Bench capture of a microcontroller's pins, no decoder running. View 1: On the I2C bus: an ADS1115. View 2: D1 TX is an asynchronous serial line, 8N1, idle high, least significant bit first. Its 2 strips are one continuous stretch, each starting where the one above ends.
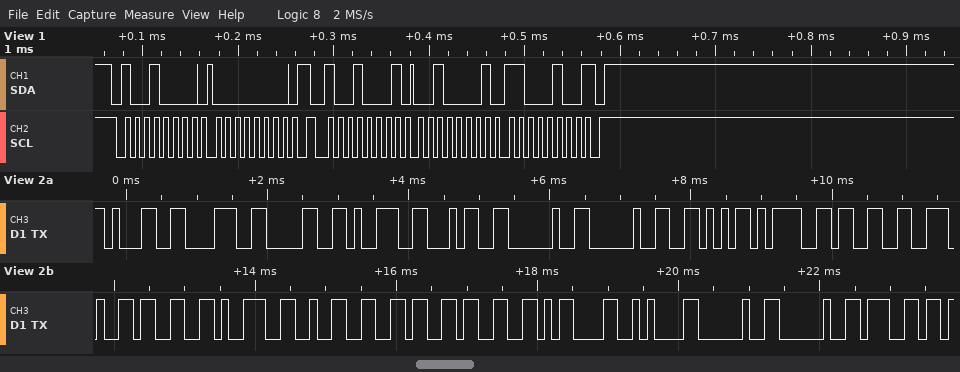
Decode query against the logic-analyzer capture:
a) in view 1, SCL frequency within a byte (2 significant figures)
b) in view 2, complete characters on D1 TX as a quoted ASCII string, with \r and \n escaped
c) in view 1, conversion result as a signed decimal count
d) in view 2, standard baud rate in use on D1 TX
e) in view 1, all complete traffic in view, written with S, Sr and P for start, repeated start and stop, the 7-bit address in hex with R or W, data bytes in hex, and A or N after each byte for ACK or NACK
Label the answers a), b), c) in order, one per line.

a) 100 kHz
b) "18094  V=3.39263\r\n  g"
c) 8644
d) 9600 baud
e) S 48W A 00 A Sr 48R A 21 A C4 N P
